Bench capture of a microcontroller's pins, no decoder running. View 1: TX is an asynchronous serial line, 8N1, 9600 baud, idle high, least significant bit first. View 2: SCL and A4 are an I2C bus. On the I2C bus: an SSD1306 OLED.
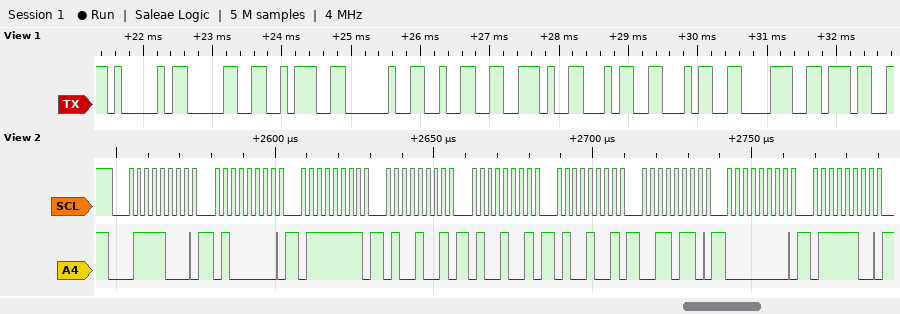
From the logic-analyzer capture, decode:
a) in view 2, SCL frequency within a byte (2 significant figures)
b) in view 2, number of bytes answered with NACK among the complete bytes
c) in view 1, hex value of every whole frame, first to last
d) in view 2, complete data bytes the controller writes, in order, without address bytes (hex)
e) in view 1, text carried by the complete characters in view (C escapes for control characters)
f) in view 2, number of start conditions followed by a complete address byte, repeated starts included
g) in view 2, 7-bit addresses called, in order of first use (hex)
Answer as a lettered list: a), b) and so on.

a) 400 kHz
b) 0
c) 41 30 3A 20 32 2E 34 34 38 37
d) 40 7F 49 49 49 36 00 7C
e) "A0: 2.4487"
f) 1
g) 0x3C
